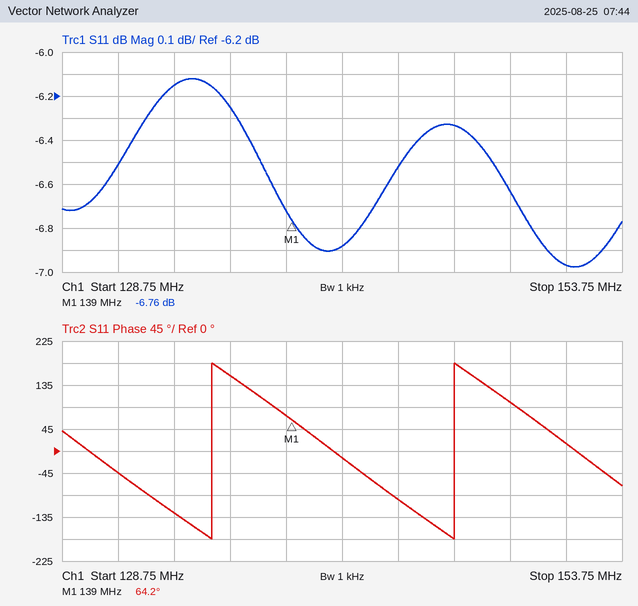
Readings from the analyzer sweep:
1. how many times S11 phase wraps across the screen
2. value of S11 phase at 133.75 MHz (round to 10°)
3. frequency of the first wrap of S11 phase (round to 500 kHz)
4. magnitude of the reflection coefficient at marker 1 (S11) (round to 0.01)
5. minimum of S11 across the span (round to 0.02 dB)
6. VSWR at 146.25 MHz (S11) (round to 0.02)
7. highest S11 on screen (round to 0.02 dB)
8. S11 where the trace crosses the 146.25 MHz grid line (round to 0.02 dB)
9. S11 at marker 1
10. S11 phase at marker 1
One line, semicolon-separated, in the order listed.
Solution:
2; -130°; 135.5 MHz; 0.46; -6.98 dB; 2.86; -6.12 dB; -6.34 dB; -6.76 dB; 64.2°
